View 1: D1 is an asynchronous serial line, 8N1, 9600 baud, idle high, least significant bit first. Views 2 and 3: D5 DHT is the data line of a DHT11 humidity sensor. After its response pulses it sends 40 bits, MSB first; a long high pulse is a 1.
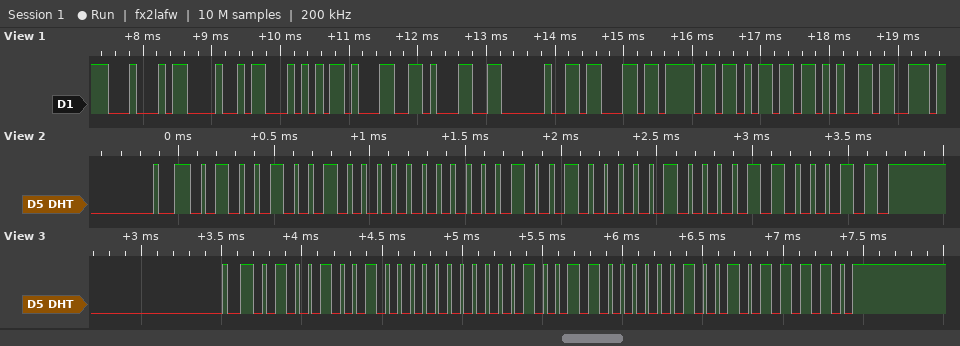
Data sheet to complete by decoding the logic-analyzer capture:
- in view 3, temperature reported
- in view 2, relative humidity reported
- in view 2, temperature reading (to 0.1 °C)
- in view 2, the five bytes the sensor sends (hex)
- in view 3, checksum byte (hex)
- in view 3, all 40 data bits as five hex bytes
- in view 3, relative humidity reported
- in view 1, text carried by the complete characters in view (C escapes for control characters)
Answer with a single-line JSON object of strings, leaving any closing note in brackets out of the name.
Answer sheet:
{"in view 3, temperature reported": "19.2 °C", "in view 2, relative humidity reported": "73 %", "in view 2, temperature reading": "18.8 °C", "in view 2, the five bytes the sensor sends": "49 00 12 08 63", "in view 3, checksum byte": "0x5E", "in view 3, all 40 data bits as five hex bytes": "49 00 13 02 5E", "in view 3, relative humidity reported": "73 %", "in view 1, text carried by the complete characters in view": "\"DHT11 come\""}
